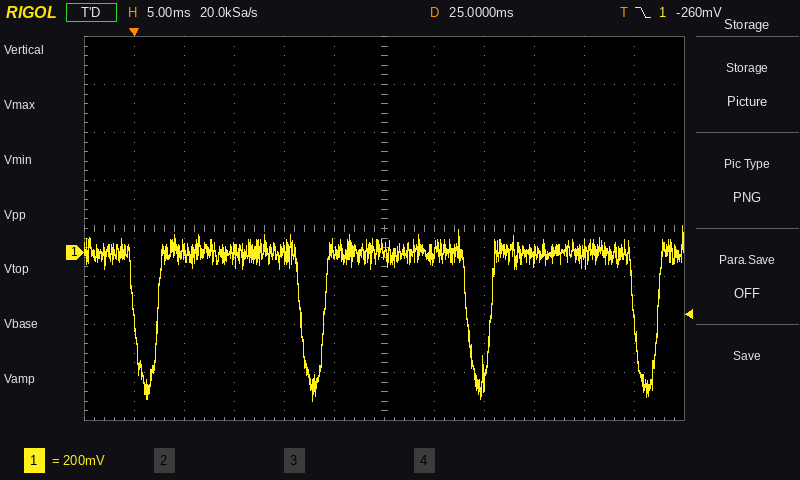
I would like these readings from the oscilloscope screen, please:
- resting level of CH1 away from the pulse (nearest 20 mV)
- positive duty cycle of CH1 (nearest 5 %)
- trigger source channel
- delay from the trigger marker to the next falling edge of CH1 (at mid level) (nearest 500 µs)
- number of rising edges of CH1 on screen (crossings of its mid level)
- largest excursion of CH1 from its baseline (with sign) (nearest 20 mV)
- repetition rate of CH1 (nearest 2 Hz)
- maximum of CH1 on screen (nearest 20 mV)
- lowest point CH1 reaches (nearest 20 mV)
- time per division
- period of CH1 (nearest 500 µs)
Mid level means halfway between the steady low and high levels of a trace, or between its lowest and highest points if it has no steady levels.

0 mV
85 %
CH1
16.5 ms
4
-620 mV
60 Hz
120 mV
-620 mV
5 ms
16.5 ms
